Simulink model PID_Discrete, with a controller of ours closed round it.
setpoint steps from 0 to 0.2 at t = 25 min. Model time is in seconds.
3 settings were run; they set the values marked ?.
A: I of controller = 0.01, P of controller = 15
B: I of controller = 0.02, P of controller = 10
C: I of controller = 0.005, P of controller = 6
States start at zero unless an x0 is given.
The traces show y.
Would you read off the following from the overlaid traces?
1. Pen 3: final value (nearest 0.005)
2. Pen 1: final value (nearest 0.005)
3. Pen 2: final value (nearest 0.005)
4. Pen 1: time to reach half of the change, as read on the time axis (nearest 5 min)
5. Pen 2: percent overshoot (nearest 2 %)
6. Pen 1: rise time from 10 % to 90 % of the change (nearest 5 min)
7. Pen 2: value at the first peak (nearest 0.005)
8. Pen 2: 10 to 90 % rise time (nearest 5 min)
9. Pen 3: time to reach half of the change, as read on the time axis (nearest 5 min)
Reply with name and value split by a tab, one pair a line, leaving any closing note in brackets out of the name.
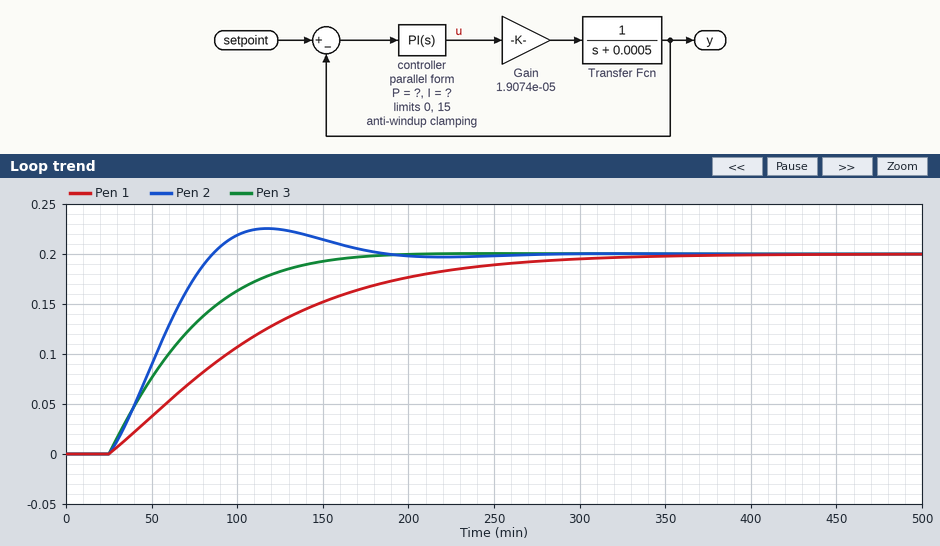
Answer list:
Pen 3: final value	0.200
Pen 1: final value	0.200
Pen 2: final value	0.200
Pen 1: time to reach half of the change, as read on the time axis	95 min
Pen 2: percent overshoot	12 %
Pen 1: rise time from 10 % to 90 % of the change	170 min
Pen 2: value at the first peak	0.225
Pen 2: 10 to 90 % rise time	45 min
Pen 3: time to reach half of the change, as read on the time axis	60 min
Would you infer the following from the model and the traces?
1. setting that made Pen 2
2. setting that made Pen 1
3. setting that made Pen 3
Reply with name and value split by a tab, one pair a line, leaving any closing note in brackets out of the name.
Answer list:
setting that made Pen 2	B
setting that made Pen 1	C
setting that made Pen 3	A
